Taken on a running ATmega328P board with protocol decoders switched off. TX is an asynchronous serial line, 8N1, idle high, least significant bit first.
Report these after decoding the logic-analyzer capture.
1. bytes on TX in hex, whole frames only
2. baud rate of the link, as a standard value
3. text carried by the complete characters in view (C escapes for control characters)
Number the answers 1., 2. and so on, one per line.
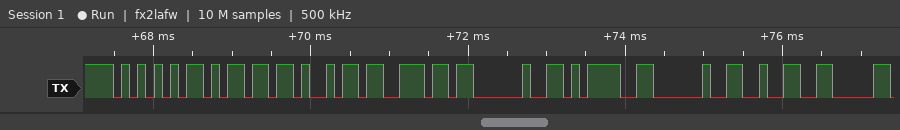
1. 0x55 0x6D 0x69 0x6E 0x20 0x3D 0x20 0x32
2. 9600 baud
3. "Umin = 2"
